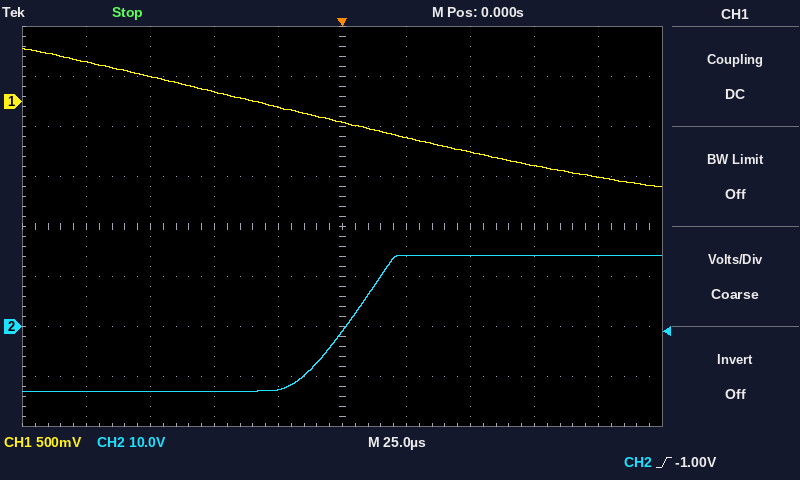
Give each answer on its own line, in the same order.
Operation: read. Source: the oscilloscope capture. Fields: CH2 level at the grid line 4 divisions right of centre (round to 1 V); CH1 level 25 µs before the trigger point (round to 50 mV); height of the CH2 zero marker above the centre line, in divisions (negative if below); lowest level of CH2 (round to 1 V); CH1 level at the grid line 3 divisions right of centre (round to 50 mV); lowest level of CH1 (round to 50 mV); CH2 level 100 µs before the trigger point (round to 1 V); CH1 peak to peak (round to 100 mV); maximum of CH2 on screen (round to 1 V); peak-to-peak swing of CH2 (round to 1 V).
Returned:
14 V
-50 mV
-2.0 div
-13 V
-650 mV
-850 mV
-13 V
1.40 V
14 V
27 V
